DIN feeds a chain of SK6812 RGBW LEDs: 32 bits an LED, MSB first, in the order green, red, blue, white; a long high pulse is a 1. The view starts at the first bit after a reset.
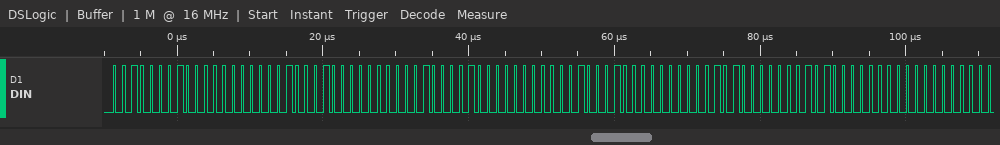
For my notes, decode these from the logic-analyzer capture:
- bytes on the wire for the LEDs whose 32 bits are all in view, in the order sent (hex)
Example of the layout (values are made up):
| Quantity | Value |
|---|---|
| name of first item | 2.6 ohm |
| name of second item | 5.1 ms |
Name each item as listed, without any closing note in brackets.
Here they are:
| Quantity | Value |
|---|---|
| bytes on the wire for the LEDs whose 32 bits are all in view, in the order sent | 21 00 11 00 21 00 11 00 28 0A 00 00 |
